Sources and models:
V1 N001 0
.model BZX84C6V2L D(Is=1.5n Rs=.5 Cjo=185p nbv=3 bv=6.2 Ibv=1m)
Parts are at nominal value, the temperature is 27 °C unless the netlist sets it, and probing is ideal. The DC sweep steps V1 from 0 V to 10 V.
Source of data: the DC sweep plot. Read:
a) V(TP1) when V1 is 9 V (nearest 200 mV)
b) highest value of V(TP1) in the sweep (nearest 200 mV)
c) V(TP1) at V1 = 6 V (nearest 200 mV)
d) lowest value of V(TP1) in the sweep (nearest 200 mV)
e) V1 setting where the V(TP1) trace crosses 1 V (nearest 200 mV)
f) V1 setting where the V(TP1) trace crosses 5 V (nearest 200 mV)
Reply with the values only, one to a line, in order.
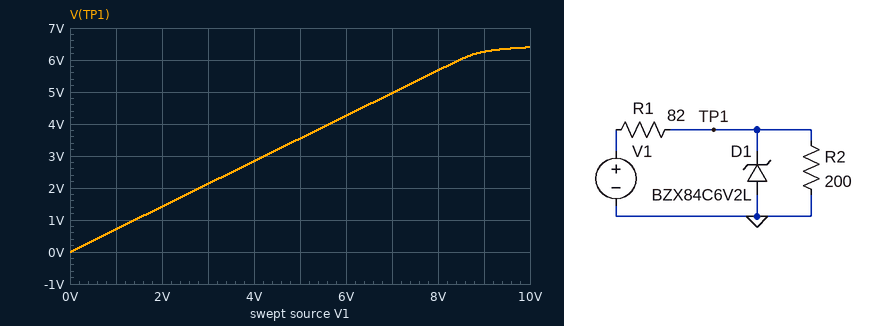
6.2 V
6.4 V
4.2 V
0 V
1.4 V
7.0 V
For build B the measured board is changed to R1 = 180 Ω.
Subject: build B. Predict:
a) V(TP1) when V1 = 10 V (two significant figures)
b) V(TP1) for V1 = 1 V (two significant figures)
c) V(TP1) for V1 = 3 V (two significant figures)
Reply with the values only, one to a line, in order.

5.3 V
530 mV
1.6 V
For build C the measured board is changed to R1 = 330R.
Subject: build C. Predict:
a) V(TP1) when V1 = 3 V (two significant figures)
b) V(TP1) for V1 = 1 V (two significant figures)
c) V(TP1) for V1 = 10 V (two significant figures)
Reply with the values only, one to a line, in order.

1.1 V
380 mV
3.8 V
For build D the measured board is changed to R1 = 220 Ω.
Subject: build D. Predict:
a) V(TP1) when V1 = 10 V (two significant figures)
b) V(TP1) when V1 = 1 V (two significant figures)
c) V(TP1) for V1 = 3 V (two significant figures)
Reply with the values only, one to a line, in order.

4.8 V
480 mV
1.4 V
